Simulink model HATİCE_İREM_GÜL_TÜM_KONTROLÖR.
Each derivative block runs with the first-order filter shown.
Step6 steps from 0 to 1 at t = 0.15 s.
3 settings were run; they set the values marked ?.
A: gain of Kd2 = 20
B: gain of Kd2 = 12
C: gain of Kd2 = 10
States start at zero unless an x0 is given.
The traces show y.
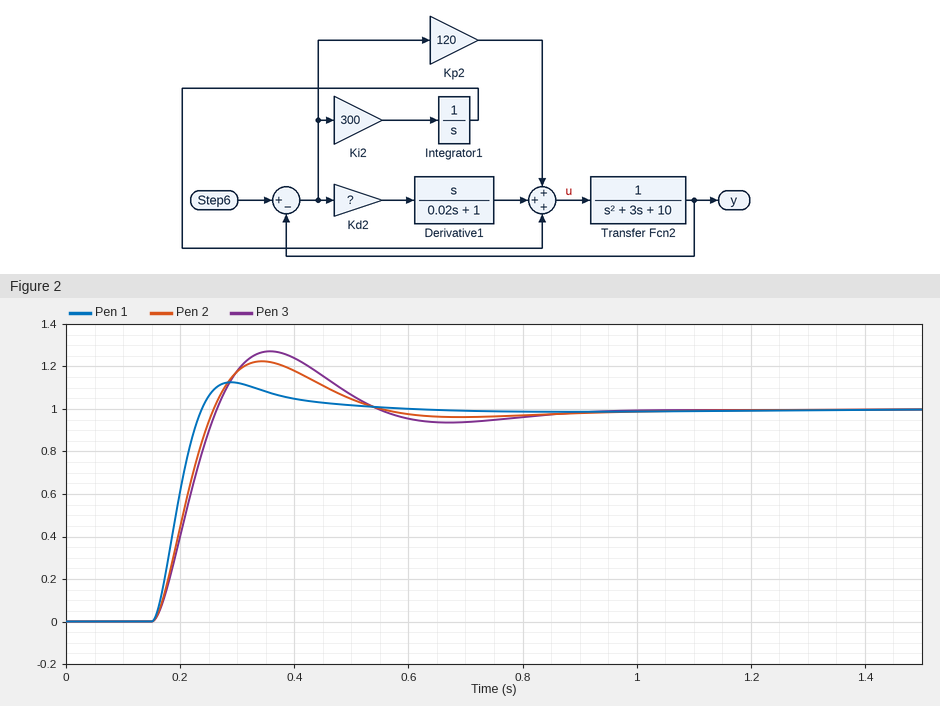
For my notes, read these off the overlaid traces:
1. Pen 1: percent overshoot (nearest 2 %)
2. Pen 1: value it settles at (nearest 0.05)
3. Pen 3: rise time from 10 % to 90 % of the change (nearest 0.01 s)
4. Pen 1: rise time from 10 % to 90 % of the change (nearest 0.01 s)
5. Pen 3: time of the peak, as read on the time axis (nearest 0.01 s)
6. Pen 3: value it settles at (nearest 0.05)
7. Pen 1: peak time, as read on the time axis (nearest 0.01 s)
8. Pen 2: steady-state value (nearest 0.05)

12 %
1.00
0.08 s
0.06 s
0.36 s
1.00
0.29 s
1.00
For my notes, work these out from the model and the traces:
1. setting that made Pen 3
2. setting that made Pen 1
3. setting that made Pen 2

C
A
B
